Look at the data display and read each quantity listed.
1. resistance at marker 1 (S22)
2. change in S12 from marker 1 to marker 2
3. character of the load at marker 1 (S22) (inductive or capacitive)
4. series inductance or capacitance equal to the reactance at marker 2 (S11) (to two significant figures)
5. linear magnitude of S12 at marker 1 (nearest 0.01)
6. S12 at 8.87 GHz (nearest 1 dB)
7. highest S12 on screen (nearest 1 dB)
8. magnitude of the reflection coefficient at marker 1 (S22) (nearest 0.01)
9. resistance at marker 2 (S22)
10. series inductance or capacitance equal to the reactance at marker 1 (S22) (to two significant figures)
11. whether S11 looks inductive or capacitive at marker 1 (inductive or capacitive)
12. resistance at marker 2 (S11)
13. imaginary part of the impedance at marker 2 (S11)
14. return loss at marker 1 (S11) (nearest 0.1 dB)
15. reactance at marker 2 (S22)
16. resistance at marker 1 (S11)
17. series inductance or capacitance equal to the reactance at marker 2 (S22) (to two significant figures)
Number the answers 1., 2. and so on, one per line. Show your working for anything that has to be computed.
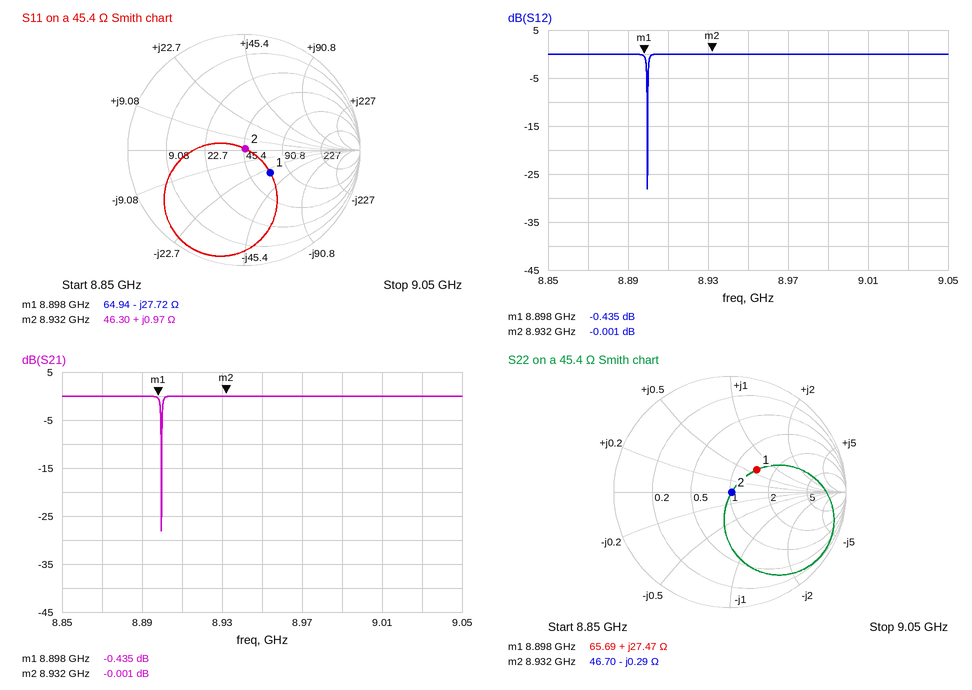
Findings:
1. 65.69 Ω
2. -0.001 − (-0.435) = 0.434 dB
3. inductive
4. L = 0.97 Ω/(2π × 8.932 GHz) ≈ 17 pH
5. 10^(-0.435/20) ≈ 0.95
6. 0 dB
7. 0 dB
8. 0.30
9. 46.70 Ω
10. L = 27.47 Ω/(2π × 8.898 GHz) ≈ 491 pH, so 490 pH to two significant figures
11. capacitive
12. 46.30 Ω
13. +0.97 Ω
14. 10.5 dB
15. -0.29 Ω
16. 64.94 Ω
17. C = 1/(2π × 8.932 GHz × 0.29 Ω) ≈ 61 pF
